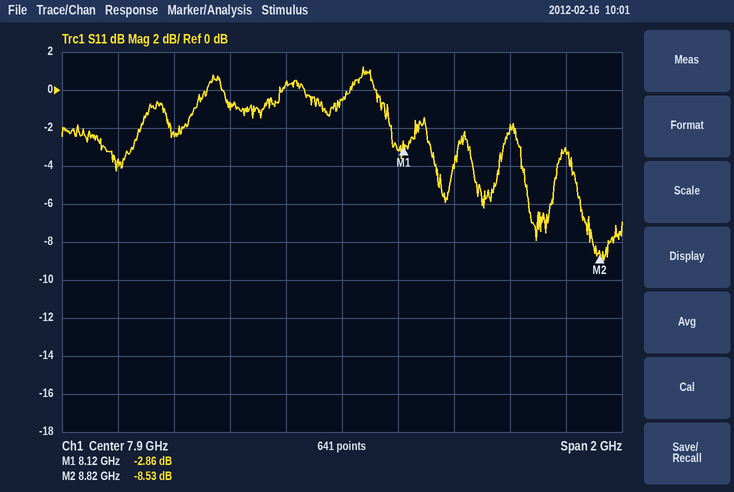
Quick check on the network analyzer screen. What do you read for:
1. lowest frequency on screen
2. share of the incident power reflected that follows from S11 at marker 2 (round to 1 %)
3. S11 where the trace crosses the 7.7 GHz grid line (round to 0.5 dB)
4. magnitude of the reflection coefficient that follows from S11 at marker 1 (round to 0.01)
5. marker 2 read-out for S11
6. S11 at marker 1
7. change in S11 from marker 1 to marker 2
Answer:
6.9 GHz
14 %
0.5 dB
0.72
-8.53 dB
-2.86 dB
-5.67 dB
